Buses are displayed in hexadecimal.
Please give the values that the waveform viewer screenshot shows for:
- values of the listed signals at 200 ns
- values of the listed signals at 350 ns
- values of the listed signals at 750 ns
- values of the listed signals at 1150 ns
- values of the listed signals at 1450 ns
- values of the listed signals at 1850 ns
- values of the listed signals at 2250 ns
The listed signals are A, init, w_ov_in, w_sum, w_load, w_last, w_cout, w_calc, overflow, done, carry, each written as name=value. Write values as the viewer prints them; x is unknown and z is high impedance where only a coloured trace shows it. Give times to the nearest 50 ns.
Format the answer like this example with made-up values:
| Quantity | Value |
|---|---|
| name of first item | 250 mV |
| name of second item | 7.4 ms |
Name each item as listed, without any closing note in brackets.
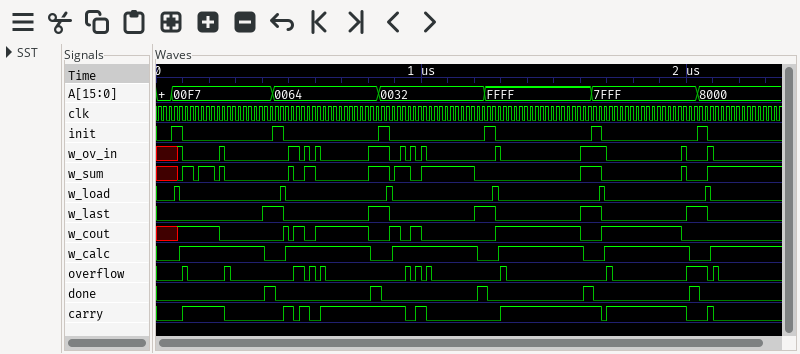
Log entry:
| Quantity | Value |
|---|---|
| values of the listed signals at 200 ns | A=00F7, init=0, w_ov_in=0, w_sum=1, w_load=0, w_last=0, w_cout=1, w_calc=1, overflow=0, done=0, carry=1 |
| values of the listed signals at 350 ns | A=00F7, init=0, w_ov_in=0, w_sum=0, w_load=0, w_last=0, w_cout=0, w_calc=1, overflow=0, done=0, carry=0 |
| values of the listed signals at 750 ns | A=0064, init=0, w_ov_in=0, w_sum=0, w_load=0, w_last=0, w_cout=1, w_calc=1, overflow=0, done=0, carry=1 |
| values of the listed signals at 1150 ns | A=0032, init=0, w_ov_in=0, w_sum=1, w_load=0, w_last=0, w_cout=0, w_calc=1, overflow=0, done=0, carry=0 |
| values of the listed signals at 1450 ns | A=FFFF, init=0, w_ov_in=0, w_sum=0, w_load=0, w_last=0, w_cout=1, w_calc=1, overflow=0, done=0, carry=1 |
| values of the listed signals at 1850 ns | A=7FFF, init=0, w_ov_in=0, w_sum=0, w_load=0, w_last=0, w_cout=1, w_calc=1, overflow=0, done=0, carry=1 |
| values of the listed signals at 2250 ns | A=8000, init=0, w_ov_in=0, w_sum=1, w_load=0, w_last=0, w_cout=0, w_calc=1, overflow=0, done=0, carry=0 |
